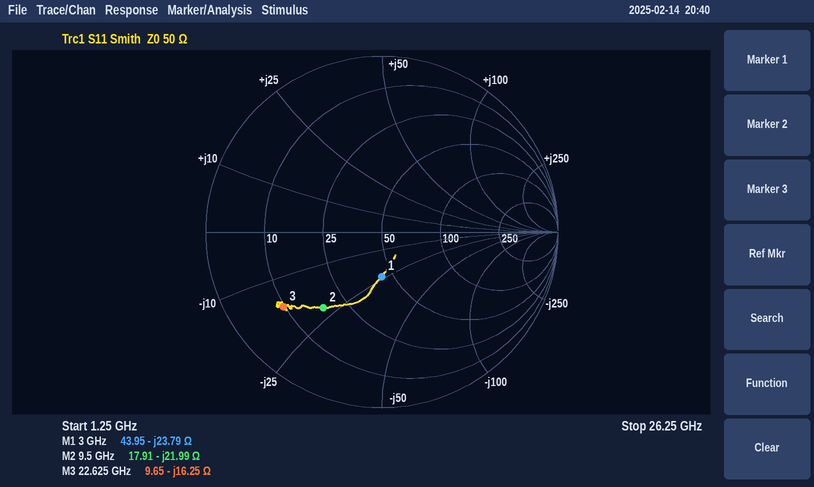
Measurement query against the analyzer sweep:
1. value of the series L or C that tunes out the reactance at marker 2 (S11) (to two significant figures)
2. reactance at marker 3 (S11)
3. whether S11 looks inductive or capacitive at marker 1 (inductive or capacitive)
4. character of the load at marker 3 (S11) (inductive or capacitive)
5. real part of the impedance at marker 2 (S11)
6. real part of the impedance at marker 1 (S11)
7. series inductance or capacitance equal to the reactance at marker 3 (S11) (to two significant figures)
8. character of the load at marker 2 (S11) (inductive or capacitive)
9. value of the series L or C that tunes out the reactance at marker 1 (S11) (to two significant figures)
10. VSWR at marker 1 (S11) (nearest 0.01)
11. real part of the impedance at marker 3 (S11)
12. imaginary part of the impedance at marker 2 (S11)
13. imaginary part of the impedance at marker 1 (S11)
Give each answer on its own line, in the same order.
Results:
370 pH
-16.25 Ω
capacitive
capacitive
17.91 Ω
43.95 Ω
430 fF
capacitive
1.3 nH
1.68
9.65 Ω
-21.99 Ω
-23.79 Ω
